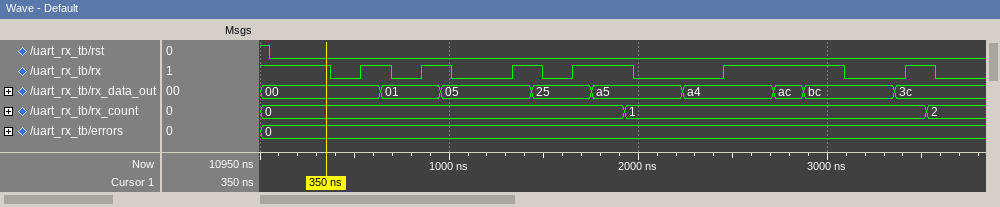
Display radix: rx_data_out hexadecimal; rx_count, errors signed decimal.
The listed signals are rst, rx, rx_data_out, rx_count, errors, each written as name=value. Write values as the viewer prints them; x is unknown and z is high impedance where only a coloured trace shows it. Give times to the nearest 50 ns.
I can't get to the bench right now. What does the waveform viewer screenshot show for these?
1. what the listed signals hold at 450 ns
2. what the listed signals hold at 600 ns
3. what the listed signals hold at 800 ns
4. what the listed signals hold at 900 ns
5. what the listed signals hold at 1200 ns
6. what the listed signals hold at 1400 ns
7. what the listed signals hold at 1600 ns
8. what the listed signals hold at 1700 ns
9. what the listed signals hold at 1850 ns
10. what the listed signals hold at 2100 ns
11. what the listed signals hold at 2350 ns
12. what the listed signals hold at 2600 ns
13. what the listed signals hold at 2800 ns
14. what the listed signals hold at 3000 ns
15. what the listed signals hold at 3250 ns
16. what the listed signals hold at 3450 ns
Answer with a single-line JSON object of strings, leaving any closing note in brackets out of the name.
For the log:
{"what the listed signals hold at 450 ns": "rst=0, rx=0, rx_data_out=00, rx_count=0, errors=0", "what the listed signals hold at 600 ns": "rst=0, rx=1, rx_data_out=00, rx_count=0, errors=0", "what the listed signals hold at 800 ns": "rst=0, rx=0, rx_data_out=01, rx_count=0, errors=0", "what the listed signals hold at 900 ns": "rst=0, rx=1, rx_data_out=01, rx_count=0, errors=0", "what the listed signals hold at 1200 ns": "rst=0, rx=0, rx_data_out=05, rx_count=0, errors=0", "what the listed signals hold at 1400 ns": "rst=0, rx=1, rx_data_out=05, rx_count=0, errors=0", "what the listed signals hold at 1600 ns": "rst=0, rx=0, rx_data_out=25, rx_count=0, errors=0", "what the listed signals hold at 1700 ns": "rst=0, rx=1, rx_data_out=25, rx_count=0, errors=0", "what the listed signals hold at 1850 ns": "rst=0, rx=1, rx_data_out=a5, rx_count=0, errors=0", "what the listed signals hold at 2100 ns": "rst=0, rx=0, rx_data_out=a5, rx_count=1, errors=0", "what the listed signals hold at 2350 ns": "rst=0, rx=0, rx_data_out=a4, rx_count=1, errors=0", "what the listed signals hold at 2600 ns": "rst=0, rx=1, rx_data_out=a4, rx_count=1, errors=0", "what the listed signals hold at 2800 ns": "rst=0, rx=1, rx_data_out=ac, rx_count=1, errors=0", "what the listed signals hold at 3000 ns": "rst=0, rx=1, rx_data_out=bc, rx_count=1, errors=0", "what the listed signals hold at 3250 ns": "rst=0, rx=0, rx_data_out=bc, rx_count=1, errors=0", "what the listed signals hold at 3450 ns": "rst=0, rx=1, rx_data_out=3c, rx_count=1, errors=0"}
